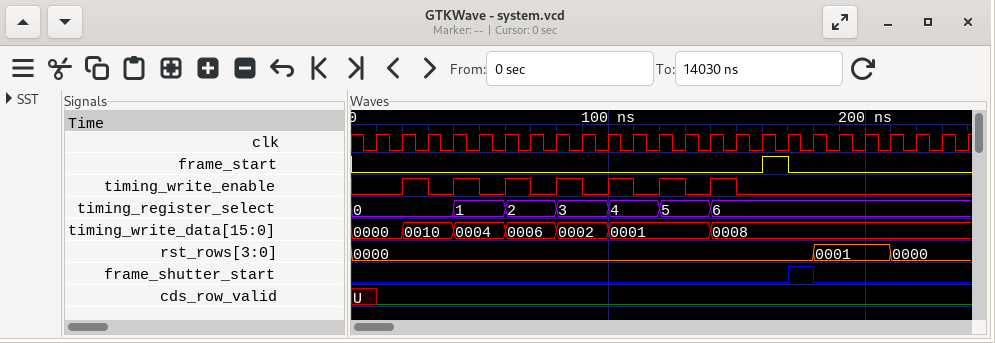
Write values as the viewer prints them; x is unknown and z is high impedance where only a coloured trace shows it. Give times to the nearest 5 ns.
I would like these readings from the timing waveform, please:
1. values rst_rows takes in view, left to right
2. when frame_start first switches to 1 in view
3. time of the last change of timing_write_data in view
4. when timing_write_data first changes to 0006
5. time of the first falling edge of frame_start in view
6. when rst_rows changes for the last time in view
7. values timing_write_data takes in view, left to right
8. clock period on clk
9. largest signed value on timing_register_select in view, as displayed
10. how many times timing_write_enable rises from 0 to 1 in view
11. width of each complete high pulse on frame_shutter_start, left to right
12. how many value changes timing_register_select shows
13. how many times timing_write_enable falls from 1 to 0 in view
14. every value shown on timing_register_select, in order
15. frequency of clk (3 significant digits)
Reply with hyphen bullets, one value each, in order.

- 0000, 0001, 0000
- 160 ns
- 140 ns
- 60 ns
- 170 ns
- 210 ns
- 0000, 0010, 0004, 0006, 0002, 0001, 0008
- 10 ns
- 6
- 7
- 10 ns
- 6
- 7
- 0, 1, 2, 3, 4, 5, 6
- 100 MHz
